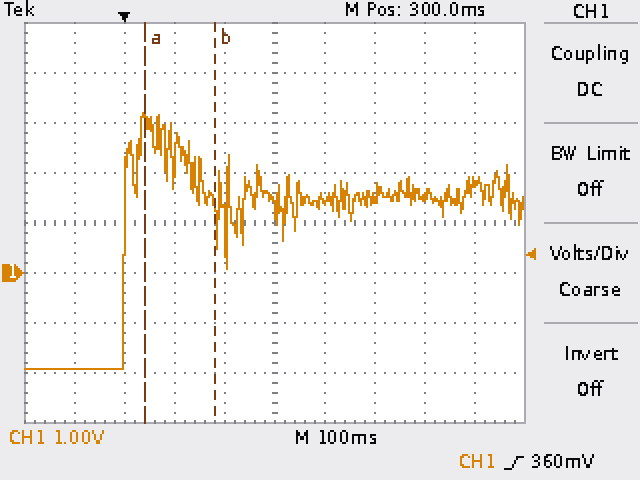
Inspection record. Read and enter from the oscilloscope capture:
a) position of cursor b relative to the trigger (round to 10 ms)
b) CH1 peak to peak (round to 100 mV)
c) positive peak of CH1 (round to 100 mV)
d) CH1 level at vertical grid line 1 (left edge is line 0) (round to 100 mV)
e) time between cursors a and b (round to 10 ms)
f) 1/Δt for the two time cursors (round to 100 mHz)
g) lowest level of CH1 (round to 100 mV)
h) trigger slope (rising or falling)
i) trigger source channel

+180 ms
5.1 V
3.2 V
-1.9 V
140 ms
7.1 Hz
-1.9 V
rising
CH1
